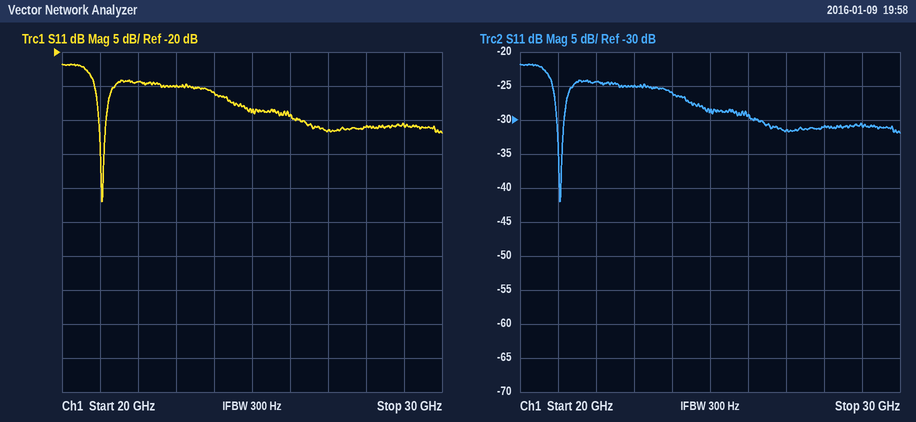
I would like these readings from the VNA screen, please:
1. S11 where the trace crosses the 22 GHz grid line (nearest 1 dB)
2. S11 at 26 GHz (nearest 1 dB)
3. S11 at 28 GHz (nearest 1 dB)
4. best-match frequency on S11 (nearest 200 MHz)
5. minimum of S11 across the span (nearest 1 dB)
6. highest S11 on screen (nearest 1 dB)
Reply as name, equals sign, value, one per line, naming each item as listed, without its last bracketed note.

S11 where the trace crosses the 22 GHz grid line = -24 dB
S11 at 26 GHz = -29 dB
S11 at 28 GHz = -31 dB
best-match frequency on S11 = 21.0 GHz
minimum of S11 across the span = -42 dB
highest S11 on screen = -22 dB
